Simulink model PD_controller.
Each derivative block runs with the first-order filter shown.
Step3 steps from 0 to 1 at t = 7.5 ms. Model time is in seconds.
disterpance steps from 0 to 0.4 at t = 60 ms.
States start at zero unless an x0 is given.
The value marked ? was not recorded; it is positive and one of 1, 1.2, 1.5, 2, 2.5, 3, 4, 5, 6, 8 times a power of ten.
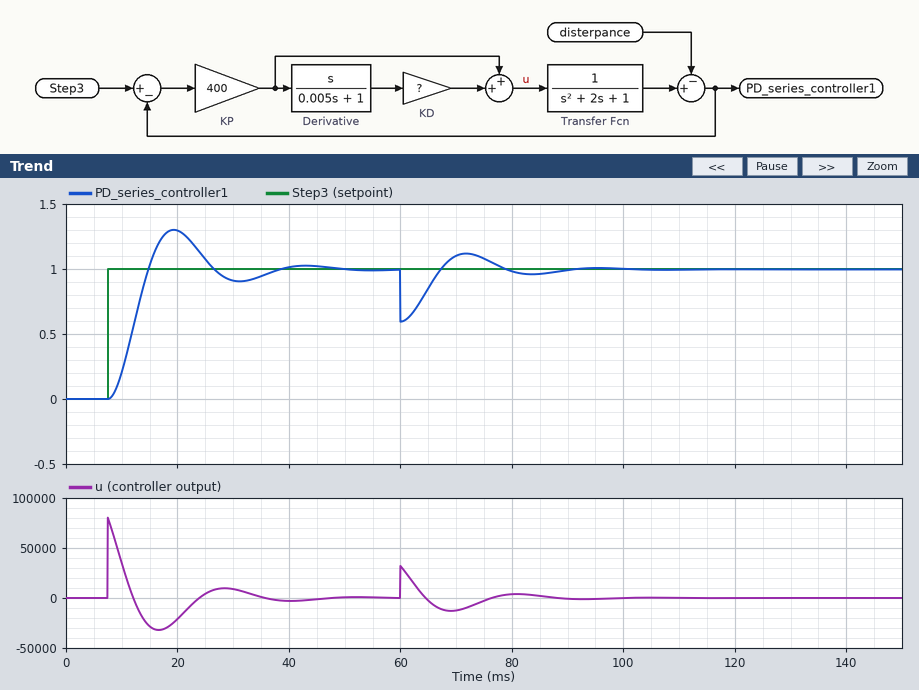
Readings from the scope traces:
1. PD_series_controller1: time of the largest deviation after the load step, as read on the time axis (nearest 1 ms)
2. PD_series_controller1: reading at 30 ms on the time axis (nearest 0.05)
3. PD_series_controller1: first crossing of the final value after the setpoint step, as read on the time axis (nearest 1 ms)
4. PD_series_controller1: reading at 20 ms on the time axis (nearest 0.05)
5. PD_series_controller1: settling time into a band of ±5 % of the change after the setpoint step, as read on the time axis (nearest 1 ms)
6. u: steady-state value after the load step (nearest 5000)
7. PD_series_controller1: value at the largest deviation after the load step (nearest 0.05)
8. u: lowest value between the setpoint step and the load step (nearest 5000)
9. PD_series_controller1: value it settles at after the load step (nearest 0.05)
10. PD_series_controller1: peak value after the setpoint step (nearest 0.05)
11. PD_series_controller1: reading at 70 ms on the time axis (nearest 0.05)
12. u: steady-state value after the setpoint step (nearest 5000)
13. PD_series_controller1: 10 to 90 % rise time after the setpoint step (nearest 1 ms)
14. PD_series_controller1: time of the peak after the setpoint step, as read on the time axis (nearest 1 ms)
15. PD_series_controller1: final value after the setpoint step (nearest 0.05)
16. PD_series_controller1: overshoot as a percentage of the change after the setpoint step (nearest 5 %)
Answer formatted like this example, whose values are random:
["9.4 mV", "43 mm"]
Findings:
["60 ms", "0.90", "15 ms", "1.30", "35 ms", "0", "0.60", "-30000", "1.00", "1.30", "1.10", "0", "5 ms", "19 ms", "1.00", "30 %"]
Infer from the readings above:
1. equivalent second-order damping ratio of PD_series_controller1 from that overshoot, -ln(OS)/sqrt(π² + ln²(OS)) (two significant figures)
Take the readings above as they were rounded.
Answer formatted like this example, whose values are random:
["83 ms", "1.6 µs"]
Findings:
["0.36"]
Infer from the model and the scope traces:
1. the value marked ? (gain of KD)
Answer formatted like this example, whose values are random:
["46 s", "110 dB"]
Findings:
["1"]
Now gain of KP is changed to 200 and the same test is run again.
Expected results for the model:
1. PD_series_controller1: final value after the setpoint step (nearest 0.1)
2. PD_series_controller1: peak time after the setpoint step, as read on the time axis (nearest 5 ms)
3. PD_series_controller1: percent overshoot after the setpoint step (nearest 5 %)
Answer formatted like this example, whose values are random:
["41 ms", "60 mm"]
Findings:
["1.0", "25 ms", "15 %"]
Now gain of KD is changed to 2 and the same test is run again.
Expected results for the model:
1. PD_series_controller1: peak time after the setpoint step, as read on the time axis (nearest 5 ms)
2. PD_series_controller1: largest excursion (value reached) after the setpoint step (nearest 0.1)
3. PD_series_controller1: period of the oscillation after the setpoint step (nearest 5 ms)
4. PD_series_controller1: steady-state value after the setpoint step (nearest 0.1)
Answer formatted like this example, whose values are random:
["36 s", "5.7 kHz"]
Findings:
["15 ms", "1.4", "15 ms", "1.0"]
